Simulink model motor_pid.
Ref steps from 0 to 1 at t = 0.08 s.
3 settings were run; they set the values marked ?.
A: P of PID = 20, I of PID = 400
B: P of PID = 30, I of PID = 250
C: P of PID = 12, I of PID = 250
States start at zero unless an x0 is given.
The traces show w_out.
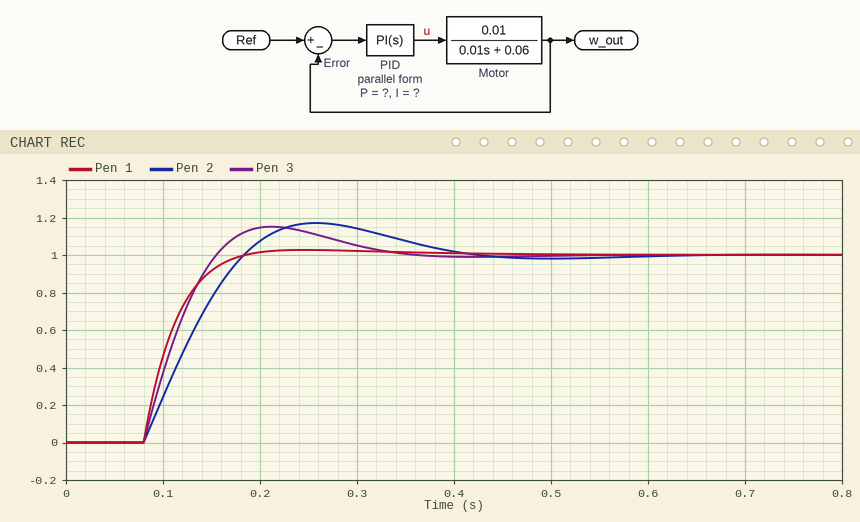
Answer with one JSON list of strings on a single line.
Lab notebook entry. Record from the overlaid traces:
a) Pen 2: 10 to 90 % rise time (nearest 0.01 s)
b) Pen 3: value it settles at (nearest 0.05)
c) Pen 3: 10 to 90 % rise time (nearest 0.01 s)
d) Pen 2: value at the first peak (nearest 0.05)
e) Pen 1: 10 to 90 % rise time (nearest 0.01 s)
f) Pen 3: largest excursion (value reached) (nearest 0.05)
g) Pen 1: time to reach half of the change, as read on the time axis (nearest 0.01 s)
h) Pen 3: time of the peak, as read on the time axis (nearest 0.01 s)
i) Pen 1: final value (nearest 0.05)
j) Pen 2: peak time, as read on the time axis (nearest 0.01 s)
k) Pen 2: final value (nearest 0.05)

["0.08 s", "1.00", "0.06 s", "1.15", "0.06 s", "1.15", "0.10 s", "0.21 s", "1.00", "0.26 s", "1.00"]
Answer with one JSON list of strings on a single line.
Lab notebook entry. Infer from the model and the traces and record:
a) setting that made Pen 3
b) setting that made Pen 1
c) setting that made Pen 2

["A", "B", "C"]
